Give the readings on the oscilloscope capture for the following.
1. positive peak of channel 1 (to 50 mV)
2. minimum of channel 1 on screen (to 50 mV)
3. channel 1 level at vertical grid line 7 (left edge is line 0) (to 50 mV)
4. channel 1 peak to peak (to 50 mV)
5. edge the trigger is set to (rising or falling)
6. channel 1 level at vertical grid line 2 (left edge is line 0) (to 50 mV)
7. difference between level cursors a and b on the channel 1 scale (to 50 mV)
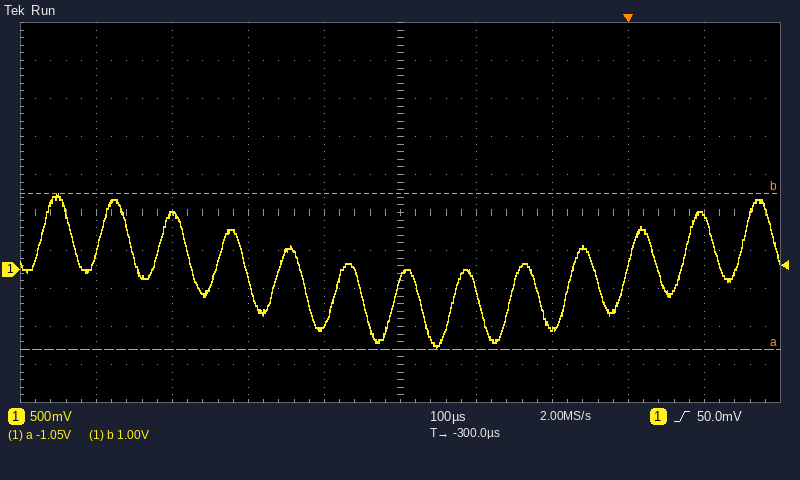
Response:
1.00 V
-1.05 V
-750 mV
2.05 V
rising
700 mV
2.05 V
